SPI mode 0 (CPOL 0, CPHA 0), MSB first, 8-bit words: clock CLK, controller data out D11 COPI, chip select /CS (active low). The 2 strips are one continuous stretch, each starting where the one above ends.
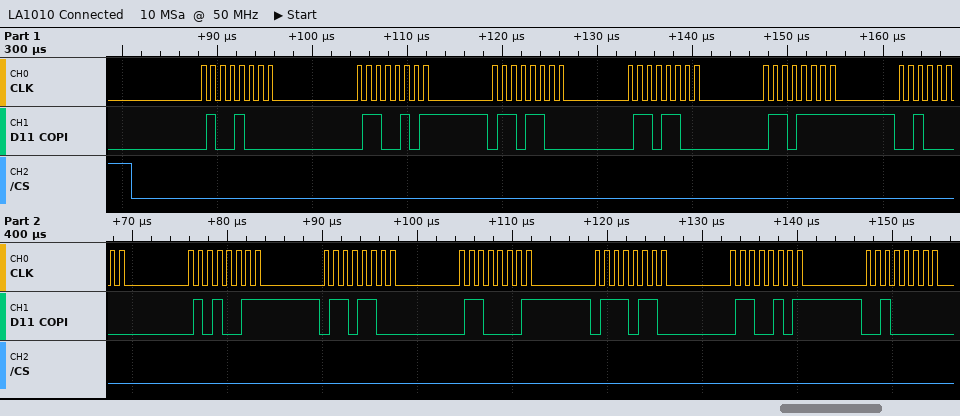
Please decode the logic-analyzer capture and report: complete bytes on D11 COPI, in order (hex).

0x48 0x65 0x6C 0x6C 0x6F 0x20 0x53 0x6C 0x61 0x76 0x65 0x20
